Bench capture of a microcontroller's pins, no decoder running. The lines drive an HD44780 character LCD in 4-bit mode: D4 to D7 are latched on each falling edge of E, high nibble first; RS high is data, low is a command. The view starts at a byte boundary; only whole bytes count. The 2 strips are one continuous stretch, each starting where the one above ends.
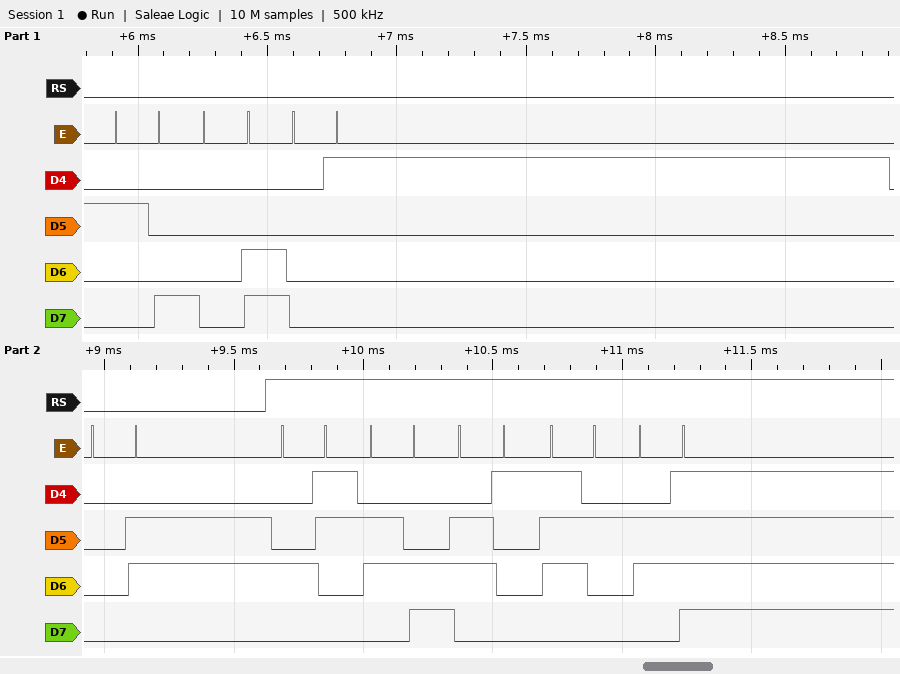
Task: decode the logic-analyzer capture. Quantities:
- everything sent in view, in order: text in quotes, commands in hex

0x28 0x0C 0x01 0x06 "Claro"
